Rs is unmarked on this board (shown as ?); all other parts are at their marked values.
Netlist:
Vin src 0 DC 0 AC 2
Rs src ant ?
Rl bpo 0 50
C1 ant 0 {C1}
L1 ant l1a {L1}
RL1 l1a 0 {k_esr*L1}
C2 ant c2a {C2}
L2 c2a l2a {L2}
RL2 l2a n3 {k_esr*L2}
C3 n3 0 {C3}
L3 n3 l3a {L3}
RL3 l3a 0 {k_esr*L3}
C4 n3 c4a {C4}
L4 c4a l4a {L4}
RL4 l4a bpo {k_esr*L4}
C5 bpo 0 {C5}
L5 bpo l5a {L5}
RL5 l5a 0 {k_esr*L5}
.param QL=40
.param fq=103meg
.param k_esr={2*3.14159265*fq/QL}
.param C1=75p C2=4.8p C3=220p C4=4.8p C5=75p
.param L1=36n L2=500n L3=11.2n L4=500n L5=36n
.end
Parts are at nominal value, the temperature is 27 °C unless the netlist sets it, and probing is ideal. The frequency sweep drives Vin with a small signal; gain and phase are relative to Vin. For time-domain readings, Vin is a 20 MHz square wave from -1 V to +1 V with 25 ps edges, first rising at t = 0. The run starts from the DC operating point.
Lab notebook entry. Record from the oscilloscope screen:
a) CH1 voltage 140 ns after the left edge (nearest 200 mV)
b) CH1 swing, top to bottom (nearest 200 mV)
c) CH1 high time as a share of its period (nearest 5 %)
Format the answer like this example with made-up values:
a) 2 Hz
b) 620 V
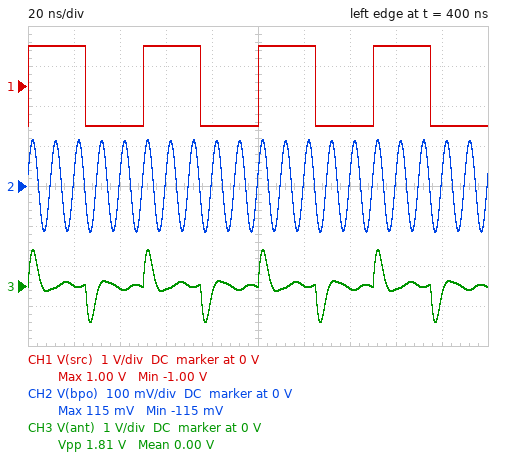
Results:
a) -1.0 V
b) 2.0 V
c) 50 %
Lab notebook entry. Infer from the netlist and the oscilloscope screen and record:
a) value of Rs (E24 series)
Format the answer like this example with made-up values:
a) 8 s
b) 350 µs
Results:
a) 27 Ω
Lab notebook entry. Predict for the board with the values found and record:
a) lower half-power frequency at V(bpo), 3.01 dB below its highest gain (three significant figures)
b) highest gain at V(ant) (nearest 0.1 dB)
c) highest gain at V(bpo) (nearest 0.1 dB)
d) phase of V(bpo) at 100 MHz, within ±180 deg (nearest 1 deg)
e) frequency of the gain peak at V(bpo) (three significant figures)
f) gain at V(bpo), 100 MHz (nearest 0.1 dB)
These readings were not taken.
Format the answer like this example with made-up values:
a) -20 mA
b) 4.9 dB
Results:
a) 91.4 MHz
b) -0.6 dB
c) -6.3 dB
d) 20 deg
e) 106 MHz
f) -7.1 dB
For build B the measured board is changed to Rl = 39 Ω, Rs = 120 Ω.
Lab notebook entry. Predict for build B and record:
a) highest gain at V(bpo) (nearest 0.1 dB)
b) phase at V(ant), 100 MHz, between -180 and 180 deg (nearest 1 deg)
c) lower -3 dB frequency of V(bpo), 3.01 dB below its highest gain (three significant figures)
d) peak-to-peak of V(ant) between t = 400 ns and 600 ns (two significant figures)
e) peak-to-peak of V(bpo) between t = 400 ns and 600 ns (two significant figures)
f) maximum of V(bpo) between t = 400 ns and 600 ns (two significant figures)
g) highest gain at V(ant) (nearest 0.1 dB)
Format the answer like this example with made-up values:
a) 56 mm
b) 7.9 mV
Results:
a) -14.5 dB
b) -24 deg
c) 90.9 MHz
d) 500 mV
e) 91 mV
f) 45 mV
g) -2.7 dB
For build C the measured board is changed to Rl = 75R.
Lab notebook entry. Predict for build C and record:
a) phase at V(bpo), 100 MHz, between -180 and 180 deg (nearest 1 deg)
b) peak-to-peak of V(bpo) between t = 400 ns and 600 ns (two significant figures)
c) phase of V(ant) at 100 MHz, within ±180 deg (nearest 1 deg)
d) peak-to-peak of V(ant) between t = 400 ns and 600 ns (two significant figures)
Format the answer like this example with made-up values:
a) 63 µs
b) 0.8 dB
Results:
a) 16 deg
b) 270 mV
c) -7 deg
d) 1.8 V
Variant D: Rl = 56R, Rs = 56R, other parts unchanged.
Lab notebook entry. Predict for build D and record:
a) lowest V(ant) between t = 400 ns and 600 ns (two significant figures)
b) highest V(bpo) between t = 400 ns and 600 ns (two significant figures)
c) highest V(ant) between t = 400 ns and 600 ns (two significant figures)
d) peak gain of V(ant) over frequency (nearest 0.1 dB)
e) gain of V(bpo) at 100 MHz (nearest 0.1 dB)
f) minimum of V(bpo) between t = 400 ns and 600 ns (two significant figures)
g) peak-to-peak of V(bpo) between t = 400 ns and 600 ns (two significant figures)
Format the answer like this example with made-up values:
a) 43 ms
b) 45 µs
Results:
a) -520 mV
b) 90 mV
c) 520 mV
d) -1.3 dB
e) -9.2 dB
f) -90 mV
g) 180 mV
